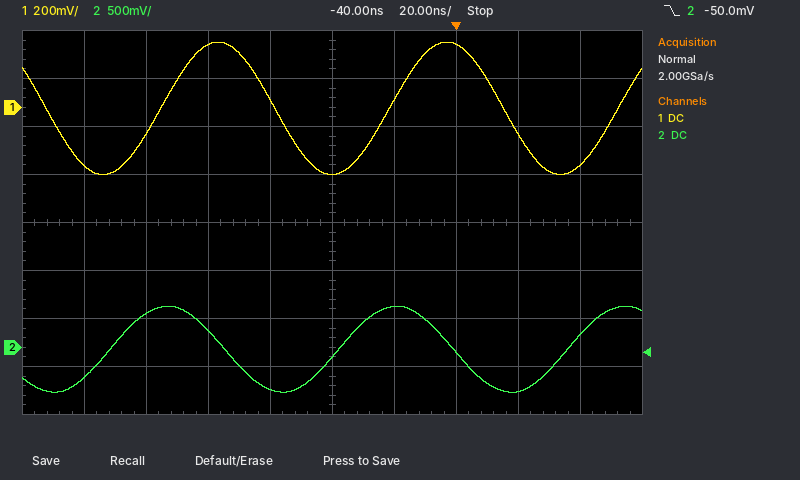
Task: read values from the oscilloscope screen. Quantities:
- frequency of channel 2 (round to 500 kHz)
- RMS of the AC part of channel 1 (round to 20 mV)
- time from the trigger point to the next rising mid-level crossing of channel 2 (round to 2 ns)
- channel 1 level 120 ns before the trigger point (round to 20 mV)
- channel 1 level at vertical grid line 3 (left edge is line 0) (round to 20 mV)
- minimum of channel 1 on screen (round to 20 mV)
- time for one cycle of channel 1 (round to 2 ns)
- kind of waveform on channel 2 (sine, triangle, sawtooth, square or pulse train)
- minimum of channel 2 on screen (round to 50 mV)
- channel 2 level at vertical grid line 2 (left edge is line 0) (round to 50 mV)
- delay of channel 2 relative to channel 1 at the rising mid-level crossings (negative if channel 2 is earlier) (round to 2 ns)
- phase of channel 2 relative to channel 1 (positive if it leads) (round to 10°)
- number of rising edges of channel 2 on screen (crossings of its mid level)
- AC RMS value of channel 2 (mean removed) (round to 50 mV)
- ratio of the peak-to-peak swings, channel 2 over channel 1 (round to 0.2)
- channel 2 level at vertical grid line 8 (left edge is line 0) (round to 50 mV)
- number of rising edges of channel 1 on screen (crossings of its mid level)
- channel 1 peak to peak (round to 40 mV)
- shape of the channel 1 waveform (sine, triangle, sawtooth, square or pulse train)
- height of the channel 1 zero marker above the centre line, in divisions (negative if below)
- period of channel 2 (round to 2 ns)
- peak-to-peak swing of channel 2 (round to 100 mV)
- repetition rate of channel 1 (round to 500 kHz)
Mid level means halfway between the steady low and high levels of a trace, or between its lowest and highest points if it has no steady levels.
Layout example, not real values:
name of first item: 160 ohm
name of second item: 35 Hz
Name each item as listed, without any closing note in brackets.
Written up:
frequency of channel 2: 13.5 MHz
RMS of the AC part of channel 1: 200 mV
time from the trigger point to the next rising mid-level crossing of channel 2: 36 ns
channel 1 level 120 ns before the trigger point: -240 mV
channel 1 level at vertical grid line 3 (left edge is line 0): 260 mV
minimum of channel 1 on screen: -280 mV
time for one cycle of channel 1: 74 ns
kind of waveform on channel 2: sine
minimum of channel 2 on screen: -450 mV
channel 2 level at vertical grid line 2 (left edge is line 0): 350 mV
delay of channel 2 relative to channel 1 at the rising mid-level crossings (negative if channel 2 is earlier): -16 ns
phase of channel 2 relative to channel 1 (positive if it leads): +80°
number of rising edges of channel 2 on screen: 3
AC RMS value of channel 2 (mean removed): 300 mV
ratio of the peak-to-peak swings, channel 2 over channel 1: 1.6
channel 2 level at vertical grid line 8 (left edge is line 0): -450 mV
number of rising edges of channel 1 on screen: 3
channel 1 peak to peak: 560 mV
shape of the channel 1 waveform: sine
height of the channel 1 zero marker above the centre line, in divisions: +2.4 div
period of channel 2: 74 ns
peak-to-peak swing of channel 2: 900 mV
repetition rate of channel 1: 13.5 MHz
